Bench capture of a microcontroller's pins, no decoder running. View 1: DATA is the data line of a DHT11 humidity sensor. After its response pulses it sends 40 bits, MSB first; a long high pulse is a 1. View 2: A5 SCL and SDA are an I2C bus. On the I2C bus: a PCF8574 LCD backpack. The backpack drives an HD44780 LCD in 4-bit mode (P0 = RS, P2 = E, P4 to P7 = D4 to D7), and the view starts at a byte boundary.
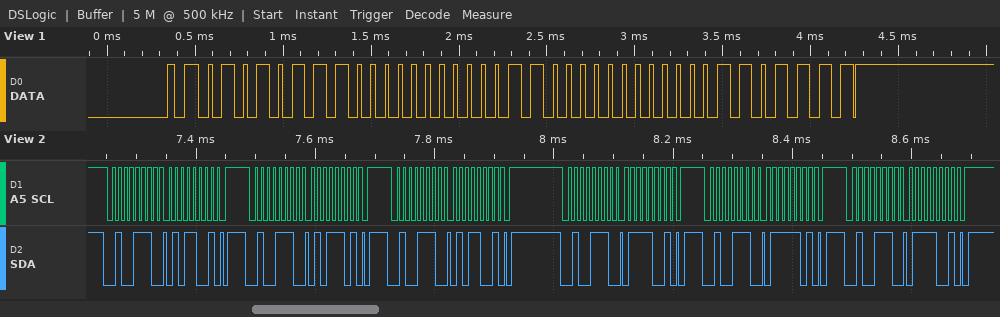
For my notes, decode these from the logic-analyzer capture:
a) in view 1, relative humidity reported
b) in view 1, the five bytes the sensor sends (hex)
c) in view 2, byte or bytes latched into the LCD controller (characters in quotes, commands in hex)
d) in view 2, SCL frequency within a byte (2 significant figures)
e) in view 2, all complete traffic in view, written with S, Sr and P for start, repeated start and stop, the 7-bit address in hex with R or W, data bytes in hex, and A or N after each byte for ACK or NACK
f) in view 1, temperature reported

87 %
57 00 18 00 6F
'W'
100 kHz
S 27W A 59 A P S 27W A 5D A P S 27W A 59 A P S 27W A 79 A P S 27W A 7D A P S 27W A 79 A P
24.0 °C
